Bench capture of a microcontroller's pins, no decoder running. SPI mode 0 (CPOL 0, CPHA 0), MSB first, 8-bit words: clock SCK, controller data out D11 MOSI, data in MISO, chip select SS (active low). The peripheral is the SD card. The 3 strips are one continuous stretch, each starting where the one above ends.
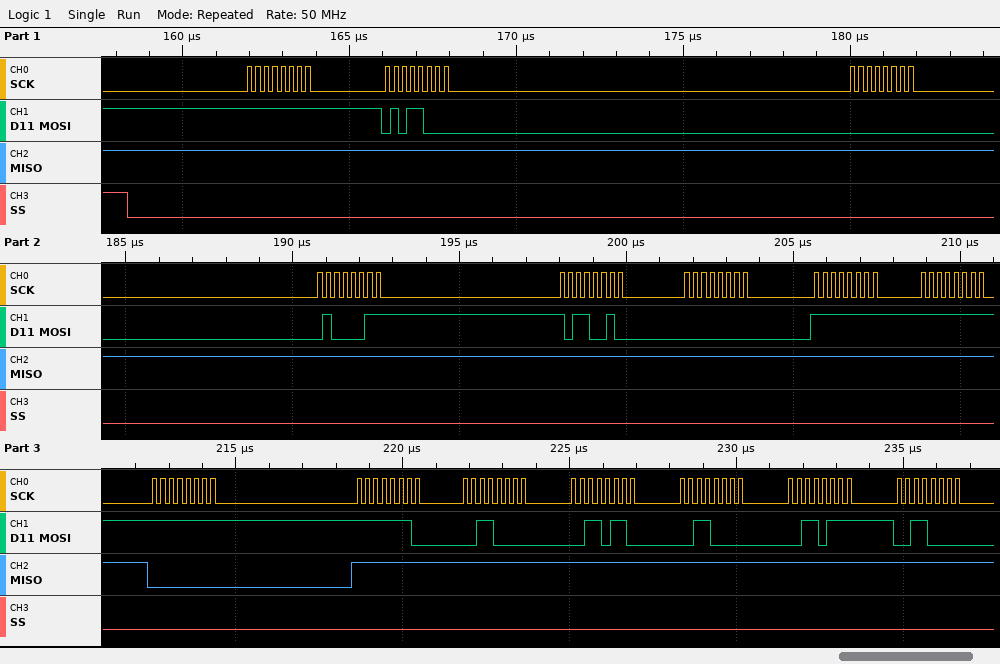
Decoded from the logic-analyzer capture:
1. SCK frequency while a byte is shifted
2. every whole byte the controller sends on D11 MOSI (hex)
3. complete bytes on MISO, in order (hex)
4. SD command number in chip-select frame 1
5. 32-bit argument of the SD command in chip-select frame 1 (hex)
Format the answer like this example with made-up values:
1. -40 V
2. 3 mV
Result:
1. 4 MHz
2. FF 58 00 43 B2 00 FF FF FF FE 30 36 30 37 30
3. FF FF FF FF FF FF FF FF 00 FF FF FF FF FF FF
4. CMD24
5. 0x0043B200
